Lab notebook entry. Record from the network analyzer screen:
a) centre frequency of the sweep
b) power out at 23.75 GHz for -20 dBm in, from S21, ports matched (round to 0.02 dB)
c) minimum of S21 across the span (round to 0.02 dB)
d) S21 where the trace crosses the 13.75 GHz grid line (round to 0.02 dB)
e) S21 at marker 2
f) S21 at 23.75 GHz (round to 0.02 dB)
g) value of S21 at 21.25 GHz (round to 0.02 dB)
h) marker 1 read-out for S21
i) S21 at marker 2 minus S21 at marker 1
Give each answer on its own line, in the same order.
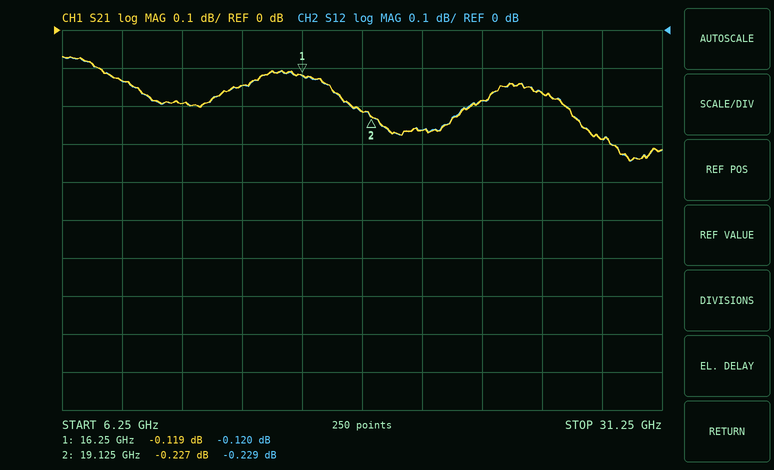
18.75 GHz
-20.18 dBm
-0.34 dB
-0.14 dB
-0.227 dB
-0.18 dB
-0.26 dB
-0.119 dB
-0.108 dB
